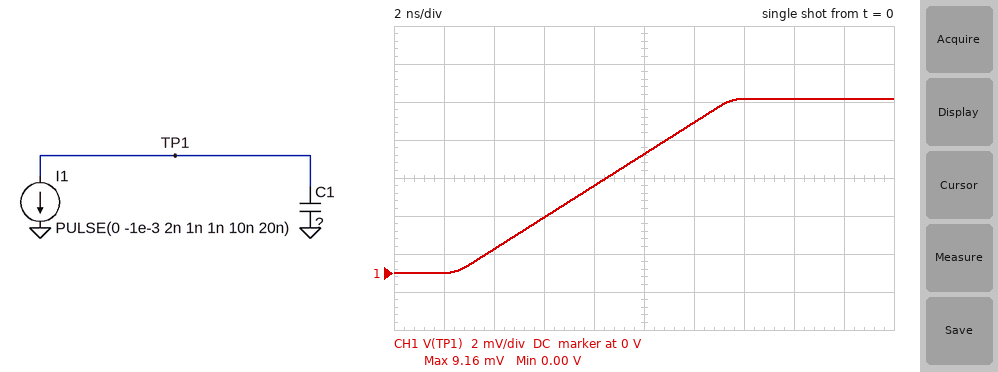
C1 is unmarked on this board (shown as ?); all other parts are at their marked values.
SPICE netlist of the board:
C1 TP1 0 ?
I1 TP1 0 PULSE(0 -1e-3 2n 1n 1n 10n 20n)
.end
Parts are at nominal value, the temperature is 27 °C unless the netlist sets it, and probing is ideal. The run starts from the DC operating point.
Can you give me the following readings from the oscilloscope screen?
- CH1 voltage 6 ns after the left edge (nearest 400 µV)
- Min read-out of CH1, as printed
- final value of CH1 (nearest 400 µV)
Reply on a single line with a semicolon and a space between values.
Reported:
2.8 mV; 0.00 V; 9.2 mV
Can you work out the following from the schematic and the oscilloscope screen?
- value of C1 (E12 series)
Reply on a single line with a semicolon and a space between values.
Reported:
1.2 nF
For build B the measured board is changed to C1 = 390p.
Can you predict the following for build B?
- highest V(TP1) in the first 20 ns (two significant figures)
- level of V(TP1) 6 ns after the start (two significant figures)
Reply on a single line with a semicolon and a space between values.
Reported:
28 mV; 9.0 mV
